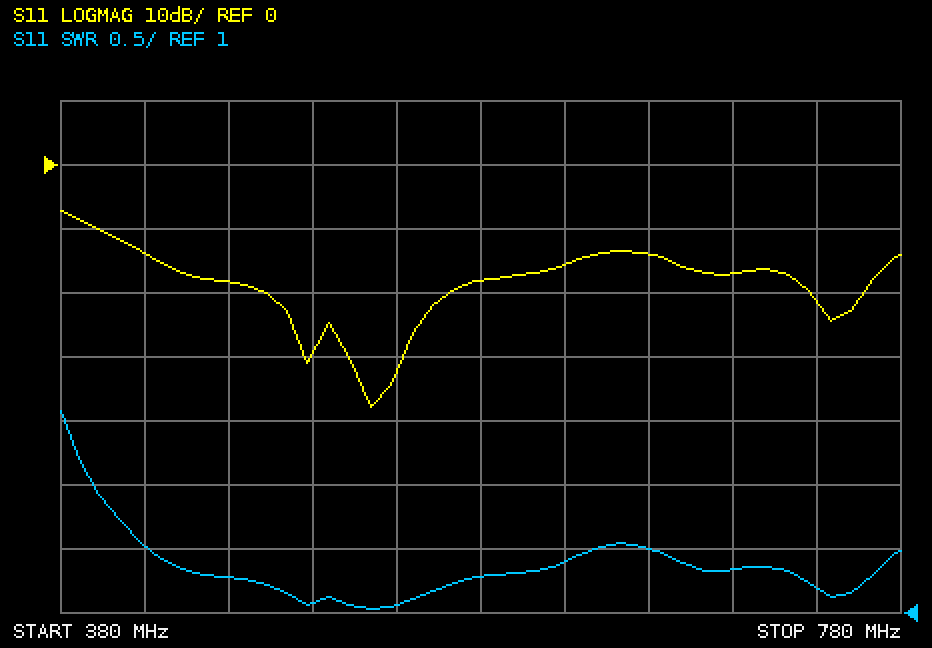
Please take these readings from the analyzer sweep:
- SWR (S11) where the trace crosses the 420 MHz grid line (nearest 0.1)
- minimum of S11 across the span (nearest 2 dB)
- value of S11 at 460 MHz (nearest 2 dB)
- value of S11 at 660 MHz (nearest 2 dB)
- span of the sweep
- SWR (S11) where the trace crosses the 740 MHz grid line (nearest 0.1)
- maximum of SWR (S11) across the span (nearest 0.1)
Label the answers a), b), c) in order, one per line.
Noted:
a) 1.5
b) -38 dB
c) -18 dB
d) -14 dB
e) 400 MHz
f) 1.2
g) 2.6
